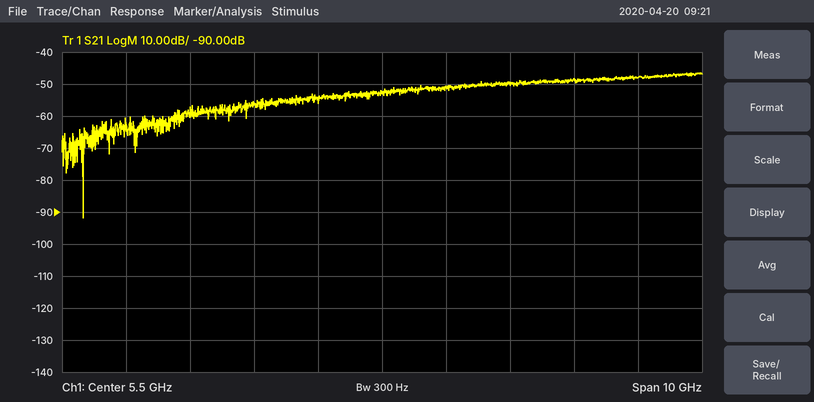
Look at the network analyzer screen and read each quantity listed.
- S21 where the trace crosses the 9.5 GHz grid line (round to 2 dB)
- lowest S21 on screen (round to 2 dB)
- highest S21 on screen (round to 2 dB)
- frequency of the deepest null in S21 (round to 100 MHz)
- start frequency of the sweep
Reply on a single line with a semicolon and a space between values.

-48 dB; -92 dB; -46 dB; 800 MHz; 500 MHz
